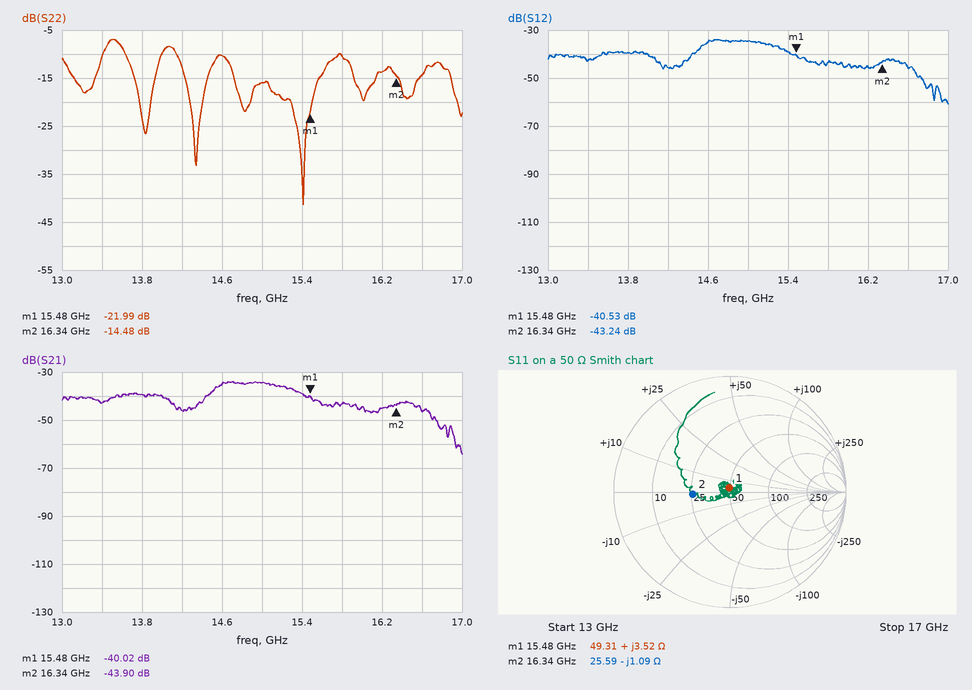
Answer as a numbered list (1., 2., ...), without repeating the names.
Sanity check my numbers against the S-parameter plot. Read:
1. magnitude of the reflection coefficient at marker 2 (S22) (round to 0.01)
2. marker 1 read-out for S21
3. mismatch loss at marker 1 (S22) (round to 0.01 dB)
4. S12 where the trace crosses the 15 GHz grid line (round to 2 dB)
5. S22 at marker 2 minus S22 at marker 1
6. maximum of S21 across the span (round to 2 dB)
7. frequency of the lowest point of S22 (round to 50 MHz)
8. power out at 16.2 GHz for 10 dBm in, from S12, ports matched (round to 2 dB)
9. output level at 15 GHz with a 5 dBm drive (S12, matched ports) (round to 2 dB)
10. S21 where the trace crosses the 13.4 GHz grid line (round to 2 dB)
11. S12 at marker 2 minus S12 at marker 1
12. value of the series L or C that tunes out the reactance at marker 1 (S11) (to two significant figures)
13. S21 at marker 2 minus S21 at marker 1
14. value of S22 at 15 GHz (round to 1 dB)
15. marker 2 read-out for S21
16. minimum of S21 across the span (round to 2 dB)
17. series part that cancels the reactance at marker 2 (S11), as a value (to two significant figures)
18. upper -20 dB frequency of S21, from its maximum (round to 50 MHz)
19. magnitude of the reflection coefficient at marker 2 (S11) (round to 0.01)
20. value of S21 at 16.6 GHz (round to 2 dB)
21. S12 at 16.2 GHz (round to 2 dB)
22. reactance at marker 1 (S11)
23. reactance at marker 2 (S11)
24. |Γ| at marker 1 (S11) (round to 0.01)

1. 0.19
2. -40.02 dB
3. 0.03 dB
4. -34 dB
5. 7.51 dB
6. -34 dB
7. 15.40 GHz
8. -36 dBm
9. -30 dBm
10. -42 dB
11. -2.71 dB
12. 2.9 pF
13. -3.88 dB
14. -16 dB
15. -43.90 dB
16. -64 dB
17. 11 pH
18. 16.85 GHz
19. 0.32
20. -46 dB
21. -46 dB
22. +3.52 Ω
23. -1.09 Ω
24. 0.04
